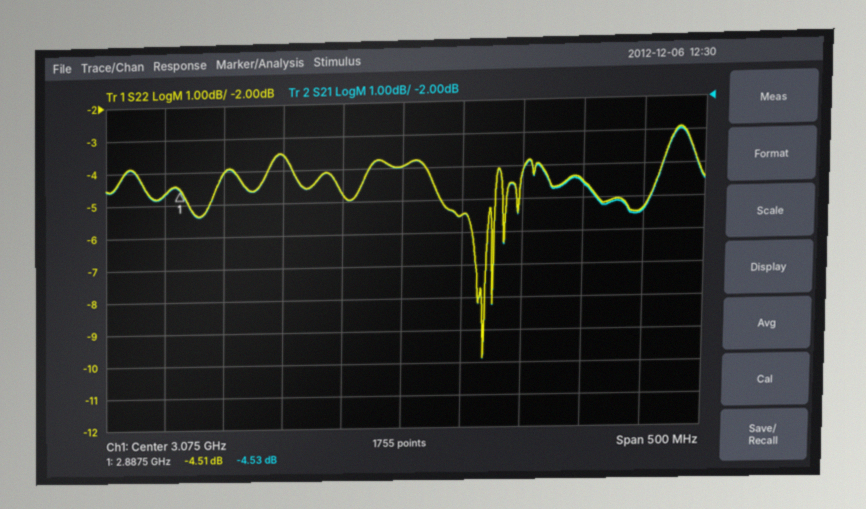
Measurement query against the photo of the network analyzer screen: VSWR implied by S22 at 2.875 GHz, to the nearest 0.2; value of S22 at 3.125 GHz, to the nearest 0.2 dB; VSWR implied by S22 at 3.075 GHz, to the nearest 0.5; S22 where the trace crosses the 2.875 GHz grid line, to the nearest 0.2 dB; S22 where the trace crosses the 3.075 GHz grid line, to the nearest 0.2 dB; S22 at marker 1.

3.8
-5.4 dB
4.5
-4.6 dB
-4.0 dB
-4.51 dB
